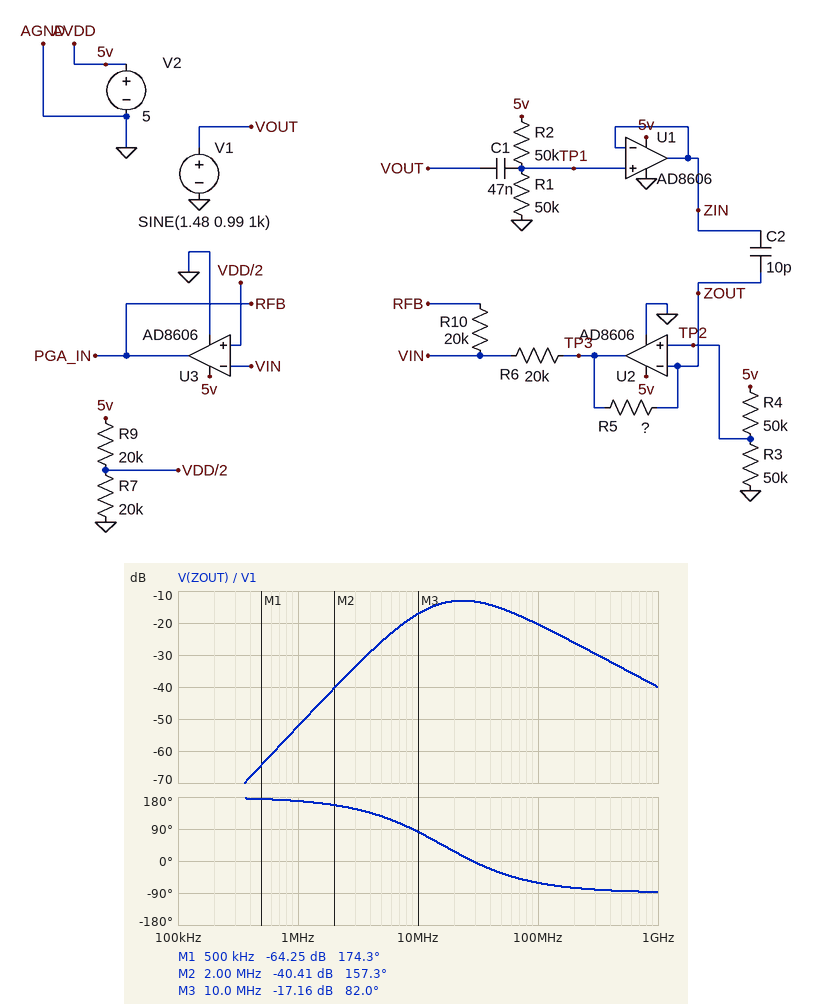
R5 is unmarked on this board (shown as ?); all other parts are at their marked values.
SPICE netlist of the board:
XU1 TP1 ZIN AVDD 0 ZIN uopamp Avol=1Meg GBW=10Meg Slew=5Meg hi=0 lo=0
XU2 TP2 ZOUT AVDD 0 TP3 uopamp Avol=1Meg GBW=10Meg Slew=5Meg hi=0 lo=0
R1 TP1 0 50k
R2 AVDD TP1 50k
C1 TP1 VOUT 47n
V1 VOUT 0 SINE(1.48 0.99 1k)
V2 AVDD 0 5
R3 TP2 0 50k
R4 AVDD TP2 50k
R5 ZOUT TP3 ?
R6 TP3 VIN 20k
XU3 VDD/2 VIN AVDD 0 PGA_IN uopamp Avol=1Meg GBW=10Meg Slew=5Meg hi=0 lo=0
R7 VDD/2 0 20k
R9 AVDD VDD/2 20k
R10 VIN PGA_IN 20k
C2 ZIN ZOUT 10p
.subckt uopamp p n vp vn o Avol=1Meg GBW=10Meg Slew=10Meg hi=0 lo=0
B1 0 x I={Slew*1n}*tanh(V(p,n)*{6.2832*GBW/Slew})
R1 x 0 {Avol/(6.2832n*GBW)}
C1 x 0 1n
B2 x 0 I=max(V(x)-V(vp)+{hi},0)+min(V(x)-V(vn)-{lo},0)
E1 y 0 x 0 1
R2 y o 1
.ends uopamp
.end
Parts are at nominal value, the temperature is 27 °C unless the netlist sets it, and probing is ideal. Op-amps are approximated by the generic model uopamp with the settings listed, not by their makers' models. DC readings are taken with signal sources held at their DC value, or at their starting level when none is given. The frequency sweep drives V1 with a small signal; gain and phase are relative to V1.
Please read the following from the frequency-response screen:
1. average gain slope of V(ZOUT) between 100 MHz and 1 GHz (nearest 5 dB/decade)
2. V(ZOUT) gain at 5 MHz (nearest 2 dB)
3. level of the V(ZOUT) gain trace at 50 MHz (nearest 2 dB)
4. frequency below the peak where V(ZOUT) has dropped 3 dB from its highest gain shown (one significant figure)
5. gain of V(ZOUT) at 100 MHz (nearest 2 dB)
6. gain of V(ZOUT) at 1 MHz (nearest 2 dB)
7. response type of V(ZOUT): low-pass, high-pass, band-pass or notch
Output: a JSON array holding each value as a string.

["-20 dB/decade", "-26 dB", "-16 dB", "10 MHz", "-20 dB", "-52 dB", "band-pass"]
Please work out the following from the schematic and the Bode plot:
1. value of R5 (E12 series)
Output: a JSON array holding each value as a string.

["390 Ω"]
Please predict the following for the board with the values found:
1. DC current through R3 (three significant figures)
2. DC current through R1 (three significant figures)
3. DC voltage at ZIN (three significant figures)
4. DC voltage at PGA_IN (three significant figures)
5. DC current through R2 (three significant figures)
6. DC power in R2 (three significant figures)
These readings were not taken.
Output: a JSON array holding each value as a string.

["50.0 µA", "50.0 µA", "2.50 V", "2.50 V", "50.0 µA", "125 µW"]
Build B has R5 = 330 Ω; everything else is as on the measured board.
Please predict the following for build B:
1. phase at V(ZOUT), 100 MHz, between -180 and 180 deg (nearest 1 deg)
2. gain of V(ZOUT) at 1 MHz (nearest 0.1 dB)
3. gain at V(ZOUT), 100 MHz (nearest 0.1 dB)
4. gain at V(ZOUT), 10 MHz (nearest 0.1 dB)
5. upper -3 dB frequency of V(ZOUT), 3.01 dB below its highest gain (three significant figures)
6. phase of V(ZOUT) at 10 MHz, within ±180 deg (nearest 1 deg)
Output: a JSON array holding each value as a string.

["-58 deg", "-53.7 dB", "-20.6 dB", "-18.8 dB", "62.2 MHz", "83 deg"]
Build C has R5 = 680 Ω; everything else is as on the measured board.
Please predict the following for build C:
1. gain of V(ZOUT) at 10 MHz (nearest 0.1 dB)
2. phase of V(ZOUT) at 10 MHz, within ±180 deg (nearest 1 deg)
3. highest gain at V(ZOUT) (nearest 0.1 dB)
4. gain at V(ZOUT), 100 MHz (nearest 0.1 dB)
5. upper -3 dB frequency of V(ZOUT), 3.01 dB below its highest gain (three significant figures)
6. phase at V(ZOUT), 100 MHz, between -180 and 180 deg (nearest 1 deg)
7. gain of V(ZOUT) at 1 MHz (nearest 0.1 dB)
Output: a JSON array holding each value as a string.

["-11.6 dB", "75 deg", "-8.7 dB", "-20.1 dB", "35.5 MHz", "-71 deg", "-47.4 dB"]
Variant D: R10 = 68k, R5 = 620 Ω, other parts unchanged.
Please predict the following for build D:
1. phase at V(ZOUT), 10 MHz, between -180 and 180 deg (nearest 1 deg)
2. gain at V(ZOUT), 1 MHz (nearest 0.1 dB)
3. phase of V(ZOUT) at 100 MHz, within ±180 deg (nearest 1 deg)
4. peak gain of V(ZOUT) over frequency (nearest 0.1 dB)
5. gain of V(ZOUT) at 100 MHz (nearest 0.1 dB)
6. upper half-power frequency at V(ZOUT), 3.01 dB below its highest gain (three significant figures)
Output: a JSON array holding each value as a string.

["76 deg", "-48.2 dB", "-70 deg", "-9.4 dB", "-20.1 dB", "38.0 MHz"]
